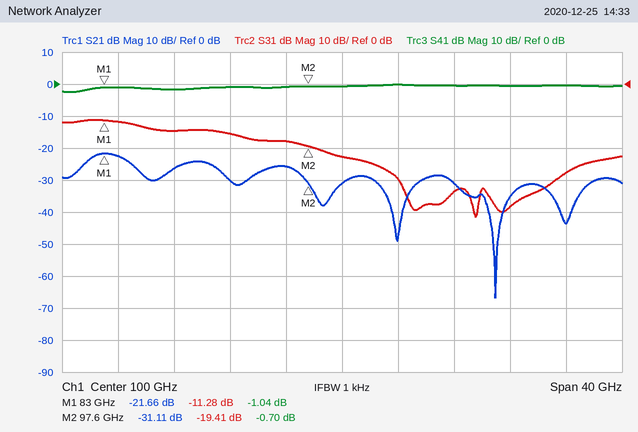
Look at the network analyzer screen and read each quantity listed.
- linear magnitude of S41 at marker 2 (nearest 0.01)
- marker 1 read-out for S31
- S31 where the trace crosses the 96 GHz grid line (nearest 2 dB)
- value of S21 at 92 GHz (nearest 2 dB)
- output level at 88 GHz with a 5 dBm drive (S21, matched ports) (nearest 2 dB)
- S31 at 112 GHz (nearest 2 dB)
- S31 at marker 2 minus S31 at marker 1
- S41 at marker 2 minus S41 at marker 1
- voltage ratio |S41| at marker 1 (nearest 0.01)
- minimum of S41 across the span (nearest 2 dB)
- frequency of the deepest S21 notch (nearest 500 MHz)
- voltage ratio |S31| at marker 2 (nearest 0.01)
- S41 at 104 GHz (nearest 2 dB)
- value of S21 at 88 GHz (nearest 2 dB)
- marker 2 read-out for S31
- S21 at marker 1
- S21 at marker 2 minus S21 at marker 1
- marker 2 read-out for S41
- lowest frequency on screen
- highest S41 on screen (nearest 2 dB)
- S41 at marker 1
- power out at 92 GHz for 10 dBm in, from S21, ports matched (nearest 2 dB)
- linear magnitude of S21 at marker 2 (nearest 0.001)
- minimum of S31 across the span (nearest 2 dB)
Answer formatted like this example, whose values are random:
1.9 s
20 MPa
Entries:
0.92
-11.28 dB
-18 dB
-30 dB
-22 dBm
-38 dB
-8.13 dB
0.34 dB
0.89
-2 dB
111.0 GHz
0.11
0 dB
-26 dB
-19.41 dB
-21.66 dB
-9.45 dB
-0.70 dB
80 GHz
0 dB
-1.04 dB
-20 dBm
0.028
-42 dB
